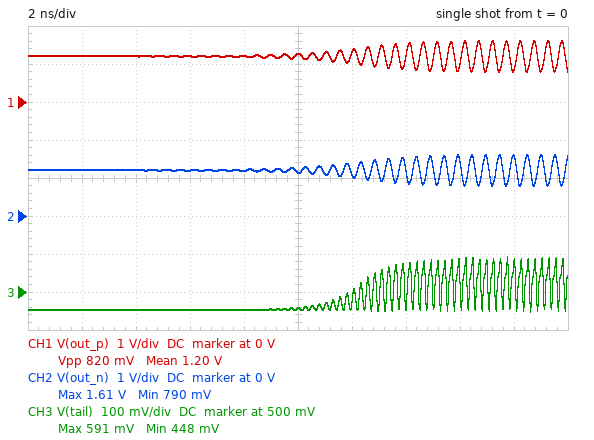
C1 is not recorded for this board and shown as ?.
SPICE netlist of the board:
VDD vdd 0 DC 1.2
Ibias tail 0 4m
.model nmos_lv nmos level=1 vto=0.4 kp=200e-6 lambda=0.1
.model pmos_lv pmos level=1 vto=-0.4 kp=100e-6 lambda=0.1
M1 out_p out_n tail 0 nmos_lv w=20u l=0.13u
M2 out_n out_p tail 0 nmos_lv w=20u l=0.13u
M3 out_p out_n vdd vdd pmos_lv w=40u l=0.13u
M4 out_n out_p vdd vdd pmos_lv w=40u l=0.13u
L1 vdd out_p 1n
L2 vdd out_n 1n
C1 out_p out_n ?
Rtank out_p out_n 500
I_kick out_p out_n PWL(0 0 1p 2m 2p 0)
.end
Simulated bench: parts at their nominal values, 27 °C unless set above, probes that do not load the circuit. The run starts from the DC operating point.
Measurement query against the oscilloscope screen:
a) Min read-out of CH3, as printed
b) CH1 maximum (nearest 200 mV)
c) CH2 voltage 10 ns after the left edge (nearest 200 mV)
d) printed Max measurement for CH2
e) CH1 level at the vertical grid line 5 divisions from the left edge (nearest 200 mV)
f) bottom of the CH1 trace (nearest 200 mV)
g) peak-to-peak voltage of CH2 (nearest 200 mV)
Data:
448 mV
1.6 V
1.2 V
1.61 V
1.2 V
800 mV
800 mV
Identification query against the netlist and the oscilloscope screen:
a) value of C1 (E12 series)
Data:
3.3 pF
